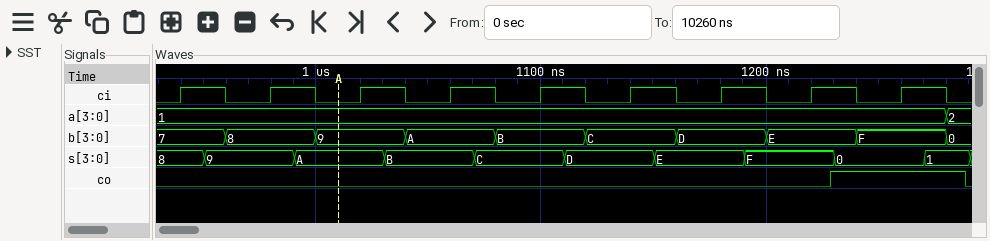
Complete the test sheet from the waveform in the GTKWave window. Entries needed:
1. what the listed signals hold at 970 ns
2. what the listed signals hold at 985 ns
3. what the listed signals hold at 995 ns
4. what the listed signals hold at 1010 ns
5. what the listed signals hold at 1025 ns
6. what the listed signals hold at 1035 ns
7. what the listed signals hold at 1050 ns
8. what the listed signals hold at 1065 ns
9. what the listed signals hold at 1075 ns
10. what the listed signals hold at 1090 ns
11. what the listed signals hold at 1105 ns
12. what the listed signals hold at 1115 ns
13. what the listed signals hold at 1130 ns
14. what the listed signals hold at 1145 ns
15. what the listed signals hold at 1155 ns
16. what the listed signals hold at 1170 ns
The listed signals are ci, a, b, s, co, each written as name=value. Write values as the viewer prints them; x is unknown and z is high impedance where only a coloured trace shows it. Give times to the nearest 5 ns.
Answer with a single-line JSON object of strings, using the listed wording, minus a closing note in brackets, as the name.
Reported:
{"what the listed signals hold at 970 ns": "ci=0, a=1, b=8, s=9, co=0", "what the listed signals hold at 985 ns": "ci=1, a=1, b=8, s=9, co=0", "what the listed signals hold at 995 ns": "ci=1, a=1, b=8, s=A, co=0", "what the listed signals hold at 1010 ns": "ci=0, a=1, b=9, s=A, co=0", "what the listed signals hold at 1025 ns": "ci=1, a=1, b=9, s=A, co=0", "what the listed signals hold at 1035 ns": "ci=1, a=1, b=9, s=B, co=0", "what the listed signals hold at 1050 ns": "ci=0, a=1, b=A, s=B, co=0", "what the listed signals hold at 1065 ns": "ci=1, a=1, b=A, s=B, co=0", "what the listed signals hold at 1075 ns": "ci=1, a=1, b=A, s=C, co=0", "what the listed signals hold at 1090 ns": "ci=0, a=1, b=B, s=C, co=0", "what the listed signals hold at 1105 ns": "ci=1, a=1, b=B, s=C, co=0", "what the listed signals hold at 1115 ns": "ci=1, a=1, b=B, s=D, co=0", "what the listed signals hold at 1130 ns": "ci=0, a=1, b=C, s=D, co=0", "what the listed signals hold at 1145 ns": "ci=1, a=1, b=C, s=D, co=0", "what the listed signals hold at 1155 ns": "ci=1, a=1, b=C, s=E, co=0", "what the listed signals hold at 1170 ns": "ci=0, a=1, b=D, s=E, co=0"}
